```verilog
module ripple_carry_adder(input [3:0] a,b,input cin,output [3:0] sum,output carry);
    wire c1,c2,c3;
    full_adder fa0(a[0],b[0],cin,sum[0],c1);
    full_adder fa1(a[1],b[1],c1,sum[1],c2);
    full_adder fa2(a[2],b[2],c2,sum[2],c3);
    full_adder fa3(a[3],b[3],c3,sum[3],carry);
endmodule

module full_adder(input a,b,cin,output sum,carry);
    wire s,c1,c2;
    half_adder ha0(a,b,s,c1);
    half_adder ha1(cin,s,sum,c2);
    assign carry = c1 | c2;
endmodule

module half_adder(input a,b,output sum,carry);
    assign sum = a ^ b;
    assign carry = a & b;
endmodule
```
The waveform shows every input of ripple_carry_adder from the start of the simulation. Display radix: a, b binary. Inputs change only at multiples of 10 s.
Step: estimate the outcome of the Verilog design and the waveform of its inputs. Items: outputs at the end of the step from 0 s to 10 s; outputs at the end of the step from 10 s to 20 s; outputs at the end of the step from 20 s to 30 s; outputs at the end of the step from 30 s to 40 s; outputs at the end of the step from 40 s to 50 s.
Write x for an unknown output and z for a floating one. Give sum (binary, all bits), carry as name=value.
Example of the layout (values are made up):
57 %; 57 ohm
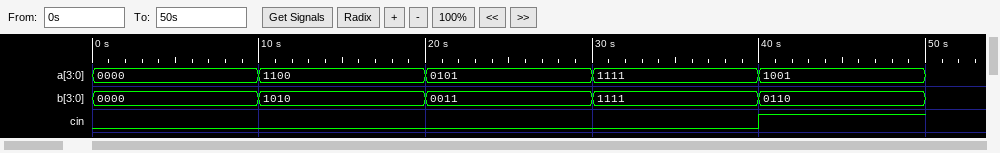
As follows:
sum=0000, carry=0; sum=0110, carry=1; sum=1000, carry=0; sum=1110, carry=1; sum=0000, carry=1
